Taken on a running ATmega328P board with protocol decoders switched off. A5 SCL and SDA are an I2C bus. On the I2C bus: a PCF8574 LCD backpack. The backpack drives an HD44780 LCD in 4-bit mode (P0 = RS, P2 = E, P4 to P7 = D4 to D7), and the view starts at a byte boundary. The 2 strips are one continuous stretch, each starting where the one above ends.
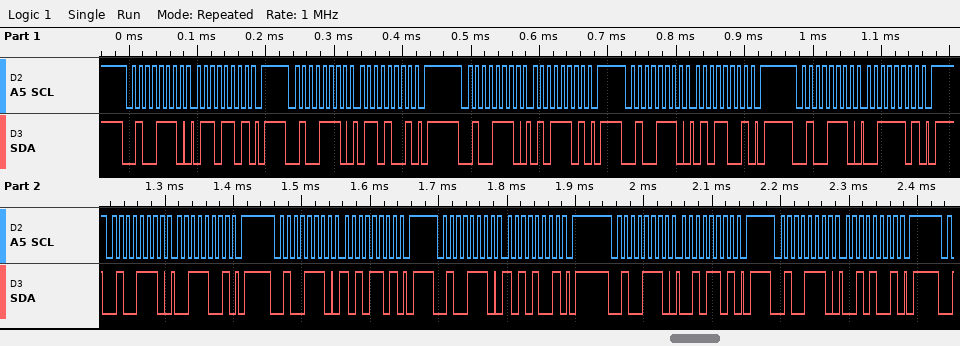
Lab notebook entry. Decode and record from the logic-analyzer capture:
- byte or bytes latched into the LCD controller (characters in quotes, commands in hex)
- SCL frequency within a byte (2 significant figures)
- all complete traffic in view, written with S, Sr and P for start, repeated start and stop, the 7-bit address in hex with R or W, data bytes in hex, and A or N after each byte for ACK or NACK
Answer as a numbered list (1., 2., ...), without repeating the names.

1. 'e' ':'
2. 100 kHz
3. S 27W A 6D A P S 27W A 69 A P S 27W A 5D A P S 27W A 59 A P S 27W A 3D A P S 27W A 39 A P S 27W A AD A P S 27W A A9 A P S 27W A 2D A P S 27W A 29 A P
